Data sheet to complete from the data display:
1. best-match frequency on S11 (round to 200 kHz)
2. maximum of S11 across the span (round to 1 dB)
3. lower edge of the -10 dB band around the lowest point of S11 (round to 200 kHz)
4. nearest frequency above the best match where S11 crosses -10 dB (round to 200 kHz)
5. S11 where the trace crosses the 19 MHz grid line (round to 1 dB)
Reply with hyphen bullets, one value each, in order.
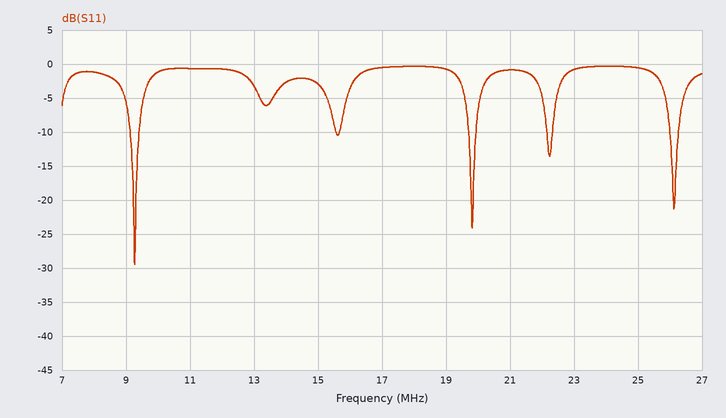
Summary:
- 9.2 MHz
- 0 dB
- 9.2 MHz
- 9.4 MHz
- -1 dB
